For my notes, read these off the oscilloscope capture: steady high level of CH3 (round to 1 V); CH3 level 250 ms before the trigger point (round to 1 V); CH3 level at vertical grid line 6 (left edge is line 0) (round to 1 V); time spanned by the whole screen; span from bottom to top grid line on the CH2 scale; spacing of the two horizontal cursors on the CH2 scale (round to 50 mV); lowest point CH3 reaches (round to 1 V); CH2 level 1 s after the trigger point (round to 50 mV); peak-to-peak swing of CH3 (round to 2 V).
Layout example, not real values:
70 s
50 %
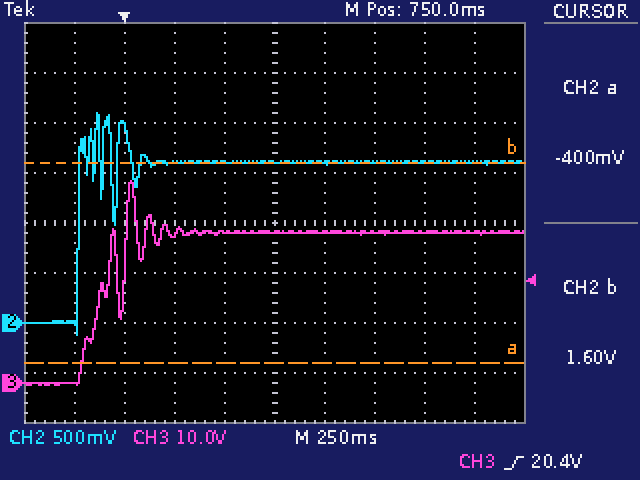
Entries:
30 V
0 V
30 V
2.5 s
4 V
2.00 V
0 V
1.60 V
40 V
